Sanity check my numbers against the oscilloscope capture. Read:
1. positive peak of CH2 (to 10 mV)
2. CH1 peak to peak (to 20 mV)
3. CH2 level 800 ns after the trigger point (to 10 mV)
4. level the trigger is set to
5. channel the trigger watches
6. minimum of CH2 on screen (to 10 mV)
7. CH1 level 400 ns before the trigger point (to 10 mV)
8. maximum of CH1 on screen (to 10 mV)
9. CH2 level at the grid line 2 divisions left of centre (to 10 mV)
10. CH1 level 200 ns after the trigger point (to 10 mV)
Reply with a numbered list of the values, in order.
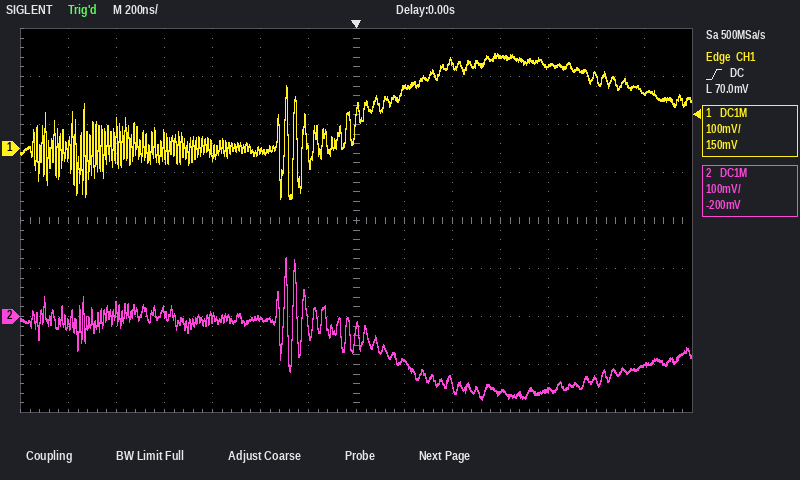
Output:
1. 120 mV
2. 300 mV
3. -150 mV
4. 70.0 mV
5. CH1
6. -170 mV
7. 0 mV
8. 200 mV
9. 0 mV
10. 130 mV
